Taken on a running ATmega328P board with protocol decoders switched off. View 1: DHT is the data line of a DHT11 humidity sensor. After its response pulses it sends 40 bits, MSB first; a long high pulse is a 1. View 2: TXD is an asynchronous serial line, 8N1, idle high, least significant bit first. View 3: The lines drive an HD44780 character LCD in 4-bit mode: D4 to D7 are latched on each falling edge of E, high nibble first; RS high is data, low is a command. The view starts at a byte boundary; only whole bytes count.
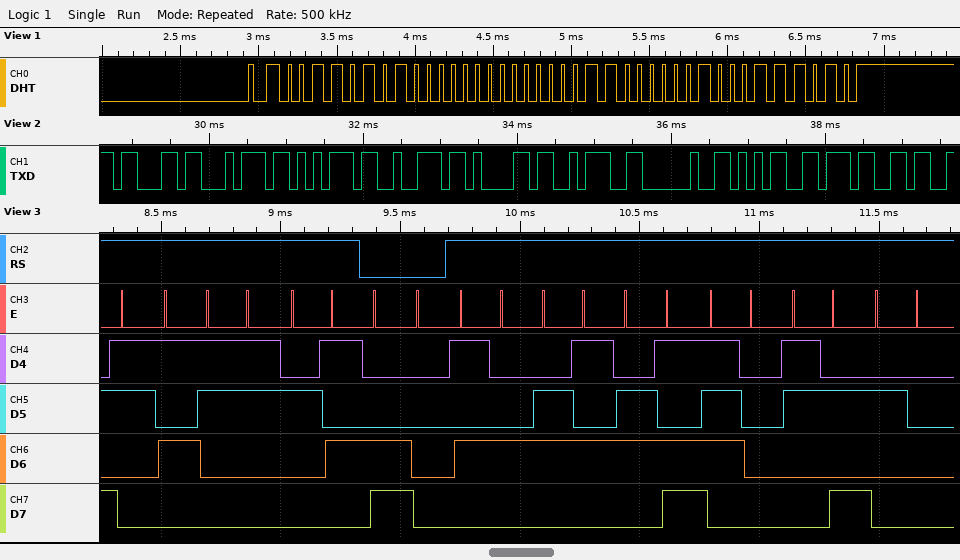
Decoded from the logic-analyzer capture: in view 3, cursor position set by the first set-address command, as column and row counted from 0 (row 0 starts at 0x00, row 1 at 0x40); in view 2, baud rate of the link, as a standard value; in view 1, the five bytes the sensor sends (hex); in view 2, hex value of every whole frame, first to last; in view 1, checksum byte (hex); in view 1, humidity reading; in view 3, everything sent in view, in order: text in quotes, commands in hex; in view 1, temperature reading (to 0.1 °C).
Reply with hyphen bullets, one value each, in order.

- column 0, row 1
- 9600 baud
- 35 00 03 02 3A
- 63 74 75 72 61 3A 20 35 37
- 0x3A
- 53 %
- "53%" 0xC0 "Temp: "
- 3.2 °C
